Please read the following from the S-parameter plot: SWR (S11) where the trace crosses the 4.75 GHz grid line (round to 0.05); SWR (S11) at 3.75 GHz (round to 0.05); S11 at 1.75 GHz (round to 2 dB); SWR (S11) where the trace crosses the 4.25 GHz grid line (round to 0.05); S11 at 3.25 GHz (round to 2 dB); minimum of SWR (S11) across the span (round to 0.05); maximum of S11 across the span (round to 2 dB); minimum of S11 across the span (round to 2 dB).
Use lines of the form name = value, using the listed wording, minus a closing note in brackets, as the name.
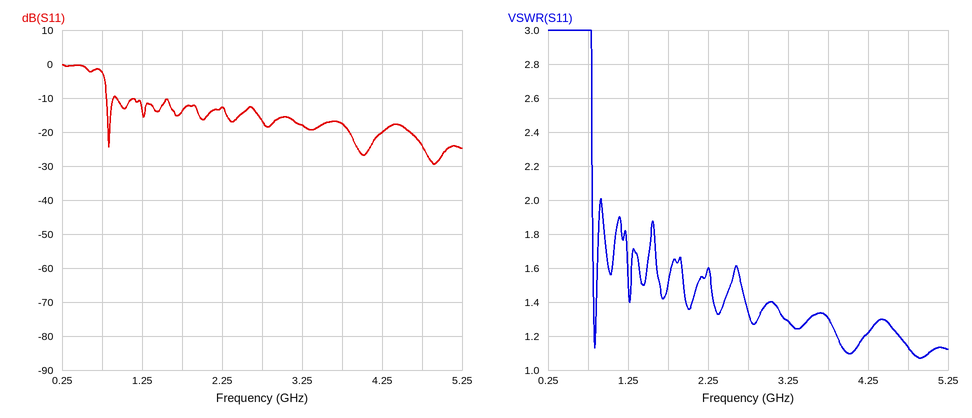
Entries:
SWR (S11) where the trace crosses the 4.75 GHz grid line = 1.15
SWR (S11) at 3.75 GHz = 1.30
S11 at 1.75 GHz = -14 dB
SWR (S11) where the trace crosses the 4.25 GHz grid line = 1.20
S11 at 3.25 GHz = -18 dB
minimum of SWR (S11) across the span = 1.05
maximum of S11 across the span = 0 dB
minimum of S11 across the span = -30 dB
